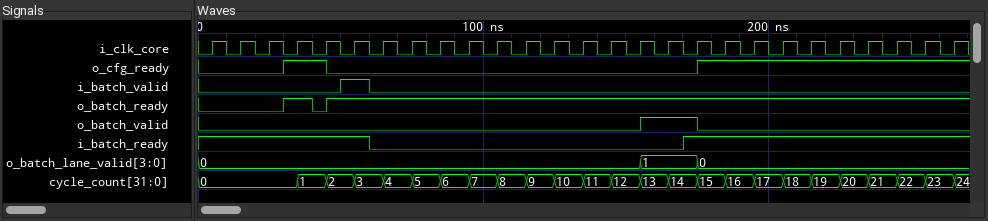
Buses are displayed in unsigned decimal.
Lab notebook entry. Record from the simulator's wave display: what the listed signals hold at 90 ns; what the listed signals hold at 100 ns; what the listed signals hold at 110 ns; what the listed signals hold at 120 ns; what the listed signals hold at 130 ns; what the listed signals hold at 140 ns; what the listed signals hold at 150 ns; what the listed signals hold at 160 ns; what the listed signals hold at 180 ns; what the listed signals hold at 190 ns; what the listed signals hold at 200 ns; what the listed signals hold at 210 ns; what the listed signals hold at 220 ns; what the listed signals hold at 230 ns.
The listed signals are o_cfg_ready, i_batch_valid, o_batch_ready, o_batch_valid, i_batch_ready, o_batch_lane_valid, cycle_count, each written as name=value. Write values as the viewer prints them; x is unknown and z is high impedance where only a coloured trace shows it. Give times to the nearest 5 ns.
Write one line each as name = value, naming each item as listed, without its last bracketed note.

what the listed signals hold at 90 ns = o_cfg_ready=0, i_batch_valid=0, o_batch_ready=1, o_batch_valid=0, i_batch_ready=0, o_batch_lane_valid=0, cycle_count=6
what the listed signals hold at 100 ns = o_cfg_ready=0, i_batch_valid=0, o_batch_ready=1, o_batch_valid=0, i_batch_ready=0, o_batch_lane_valid=0, cycle_count=7
what the listed signals hold at 110 ns = o_cfg_ready=0, i_batch_valid=0, o_batch_ready=1, o_batch_valid=0, i_batch_ready=0, o_batch_lane_valid=0, cycle_count=8
what the listed signals hold at 120 ns = o_cfg_ready=0, i_batch_valid=0, o_batch_ready=1, o_batch_valid=0, i_batch_ready=0, o_batch_lane_valid=0, cycle_count=9
what the listed signals hold at 130 ns = o_cfg_ready=0, i_batch_valid=0, o_batch_ready=1, o_batch_valid=0, i_batch_ready=0, o_batch_lane_valid=0, cycle_count=10
what the listed signals hold at 140 ns = o_cfg_ready=0, i_batch_valid=0, o_batch_ready=1, o_batch_valid=0, i_batch_ready=0, o_batch_lane_valid=0, cycle_count=11
what the listed signals hold at 150 ns = o_cfg_ready=0, i_batch_valid=0, o_batch_ready=1, o_batch_valid=0, i_batch_ready=0, o_batch_lane_valid=0, cycle_count=12
what the listed signals hold at 160 ns = o_cfg_ready=0, i_batch_valid=0, o_batch_ready=1, o_batch_valid=1, i_batch_ready=0, o_batch_lane_valid=1, cycle_count=13
what the listed signals hold at 180 ns = o_cfg_ready=1, i_batch_valid=0, o_batch_ready=1, o_batch_valid=0, i_batch_ready=1, o_batch_lane_valid=0, cycle_count=15
what the listed signals hold at 190 ns = o_cfg_ready=1, i_batch_valid=0, o_batch_ready=1, o_batch_valid=0, i_batch_ready=1, o_batch_lane_valid=0, cycle_count=16
what the listed signals hold at 200 ns = o_cfg_ready=1, i_batch_valid=0, o_batch_ready=1, o_batch_valid=0, i_batch_ready=1, o_batch_lane_valid=0, cycle_count=17
what the listed signals hold at 210 ns = o_cfg_ready=1, i_batch_valid=0, o_batch_ready=1, o_batch_valid=0, i_batch_ready=1, o_batch_lane_valid=0, cycle_count=18
what the listed signals hold at 220 ns = o_cfg_ready=1, i_batch_valid=0, o_batch_ready=1, o_batch_valid=0, i_batch_ready=1, o_batch_lane_valid=0, cycle_count=19
what the listed signals hold at 230 ns = o_cfg_ready=1, i_batch_valid=0, o_batch_ready=1, o_batch_valid=0, i_batch_ready=1, o_batch_lane_valid=0, cycle_count=20
